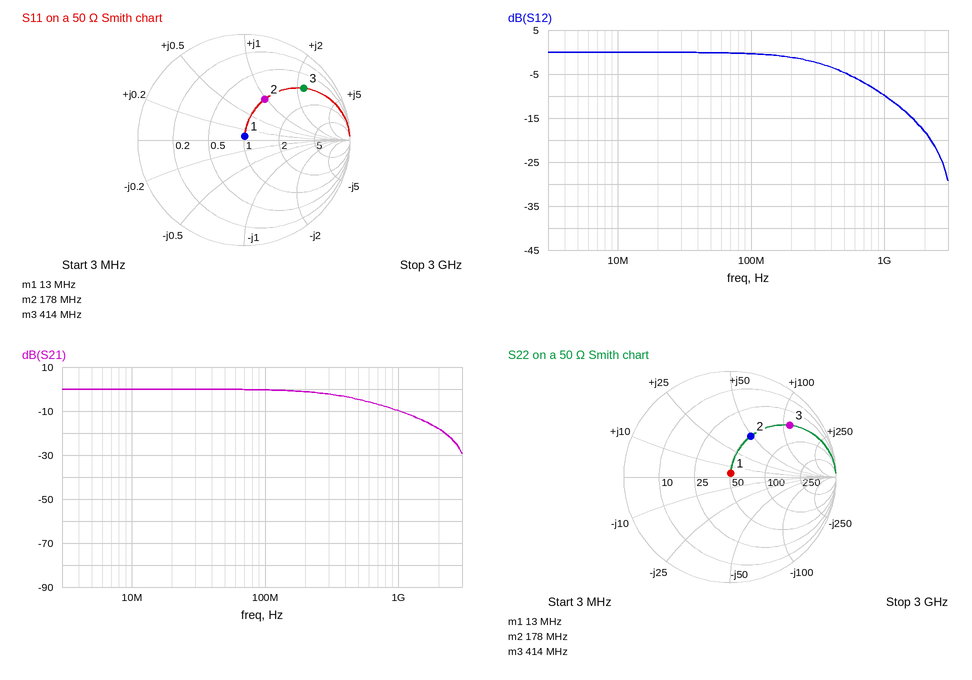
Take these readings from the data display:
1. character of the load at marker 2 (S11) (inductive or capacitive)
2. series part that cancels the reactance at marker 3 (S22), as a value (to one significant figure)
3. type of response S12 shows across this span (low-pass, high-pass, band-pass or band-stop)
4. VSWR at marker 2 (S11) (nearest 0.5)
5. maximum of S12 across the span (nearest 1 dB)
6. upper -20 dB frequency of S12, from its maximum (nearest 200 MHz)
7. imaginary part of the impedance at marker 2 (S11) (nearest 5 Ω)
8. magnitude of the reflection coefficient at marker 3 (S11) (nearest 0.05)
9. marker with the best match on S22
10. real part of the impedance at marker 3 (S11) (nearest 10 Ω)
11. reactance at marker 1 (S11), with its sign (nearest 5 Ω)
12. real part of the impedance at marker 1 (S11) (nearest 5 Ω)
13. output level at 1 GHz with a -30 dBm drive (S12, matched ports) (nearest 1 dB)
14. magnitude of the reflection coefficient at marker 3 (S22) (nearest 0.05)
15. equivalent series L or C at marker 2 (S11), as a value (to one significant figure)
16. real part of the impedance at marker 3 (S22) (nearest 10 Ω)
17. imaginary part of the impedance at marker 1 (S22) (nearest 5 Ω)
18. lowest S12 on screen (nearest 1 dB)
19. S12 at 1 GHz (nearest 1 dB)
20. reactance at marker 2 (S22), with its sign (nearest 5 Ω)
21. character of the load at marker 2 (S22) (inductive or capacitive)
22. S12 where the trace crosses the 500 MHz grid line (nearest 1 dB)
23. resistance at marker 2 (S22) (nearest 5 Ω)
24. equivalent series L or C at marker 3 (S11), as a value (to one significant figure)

inductive
3 pF
low-pass
2.5
0 dB
2.2 GHz
+50 Ω
0.75
marker 1
50 Ω
+5 Ω
50 Ω
-40 dBm
0.75
40 nH
50 Ω
+5 Ω
-29 dB
-10 dB
+50 Ω
inductive
-5 dB
50 Ω
40 nH
